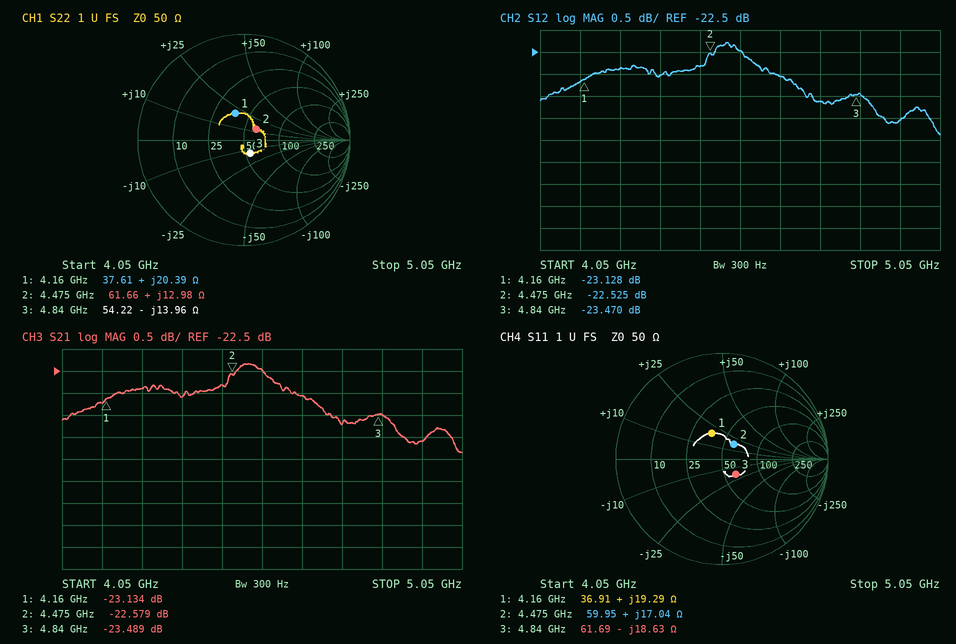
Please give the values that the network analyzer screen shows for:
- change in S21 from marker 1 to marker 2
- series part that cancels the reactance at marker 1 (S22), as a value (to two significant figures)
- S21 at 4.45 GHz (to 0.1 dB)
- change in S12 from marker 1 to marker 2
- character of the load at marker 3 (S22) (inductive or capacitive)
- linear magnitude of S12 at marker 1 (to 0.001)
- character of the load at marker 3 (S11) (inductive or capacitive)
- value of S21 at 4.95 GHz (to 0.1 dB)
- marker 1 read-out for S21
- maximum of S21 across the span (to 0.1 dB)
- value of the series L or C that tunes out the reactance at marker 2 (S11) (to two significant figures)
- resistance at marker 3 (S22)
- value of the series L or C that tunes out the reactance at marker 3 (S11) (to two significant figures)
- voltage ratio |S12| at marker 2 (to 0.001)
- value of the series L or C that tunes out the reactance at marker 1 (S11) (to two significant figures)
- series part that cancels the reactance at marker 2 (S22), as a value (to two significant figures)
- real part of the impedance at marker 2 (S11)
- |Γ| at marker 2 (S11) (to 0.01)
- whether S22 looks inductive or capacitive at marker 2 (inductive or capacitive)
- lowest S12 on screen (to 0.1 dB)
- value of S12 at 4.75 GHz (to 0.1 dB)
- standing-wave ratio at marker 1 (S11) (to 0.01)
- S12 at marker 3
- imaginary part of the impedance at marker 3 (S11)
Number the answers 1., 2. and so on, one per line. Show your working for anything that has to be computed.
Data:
1. -22.579 − (-23.134) = 0.555 dB
2. C = 1/(2π × 4.16 GHz × 20.39 Ω) ≈ 1.9 pF
3. -22.8 dB
4. -22.525 − (-23.128) = 0.603 dB
5. capacitive
6. 10^(-23.128/20) ≈ 0.070
7. capacitive
8. -24.1 dB
9. -23.134 dB
10. -22.3 dB
11. C = 1/(2π × 4.475 GHz × 17.04 Ω) ≈ 2.1 pF
12. 54.22 Ω
13. L = 18.63 Ω/(2π × 4.84 GHz) ≈ 613 pH, so 610 pH to two significant figures
14. 10^(-22.525/20) ≈ 0.075
15. C = 1/(2π × 4.16 GHz × 19.29 Ω) ≈ 2.0 pF
16. C = 1/(2π × 4.475 GHz × 12.98 Ω) ≈ 2.7 pF
17. 59.95 Ω
18. 0.18
19. inductive
20. -24.4 dB
21. -23.6 dB
22. 1.71
23. -23.470 dB
24. -18.63 Ω
